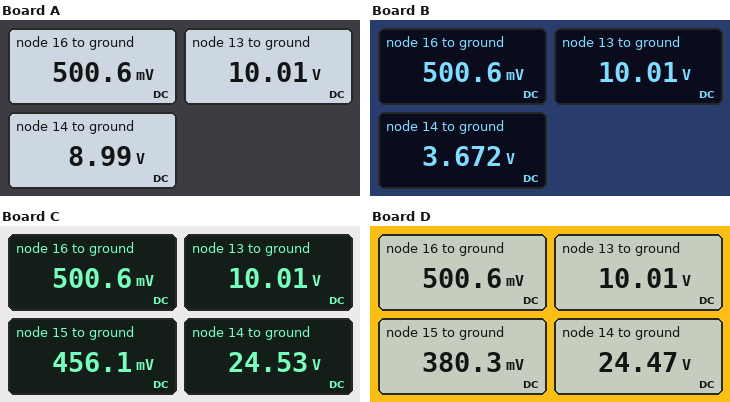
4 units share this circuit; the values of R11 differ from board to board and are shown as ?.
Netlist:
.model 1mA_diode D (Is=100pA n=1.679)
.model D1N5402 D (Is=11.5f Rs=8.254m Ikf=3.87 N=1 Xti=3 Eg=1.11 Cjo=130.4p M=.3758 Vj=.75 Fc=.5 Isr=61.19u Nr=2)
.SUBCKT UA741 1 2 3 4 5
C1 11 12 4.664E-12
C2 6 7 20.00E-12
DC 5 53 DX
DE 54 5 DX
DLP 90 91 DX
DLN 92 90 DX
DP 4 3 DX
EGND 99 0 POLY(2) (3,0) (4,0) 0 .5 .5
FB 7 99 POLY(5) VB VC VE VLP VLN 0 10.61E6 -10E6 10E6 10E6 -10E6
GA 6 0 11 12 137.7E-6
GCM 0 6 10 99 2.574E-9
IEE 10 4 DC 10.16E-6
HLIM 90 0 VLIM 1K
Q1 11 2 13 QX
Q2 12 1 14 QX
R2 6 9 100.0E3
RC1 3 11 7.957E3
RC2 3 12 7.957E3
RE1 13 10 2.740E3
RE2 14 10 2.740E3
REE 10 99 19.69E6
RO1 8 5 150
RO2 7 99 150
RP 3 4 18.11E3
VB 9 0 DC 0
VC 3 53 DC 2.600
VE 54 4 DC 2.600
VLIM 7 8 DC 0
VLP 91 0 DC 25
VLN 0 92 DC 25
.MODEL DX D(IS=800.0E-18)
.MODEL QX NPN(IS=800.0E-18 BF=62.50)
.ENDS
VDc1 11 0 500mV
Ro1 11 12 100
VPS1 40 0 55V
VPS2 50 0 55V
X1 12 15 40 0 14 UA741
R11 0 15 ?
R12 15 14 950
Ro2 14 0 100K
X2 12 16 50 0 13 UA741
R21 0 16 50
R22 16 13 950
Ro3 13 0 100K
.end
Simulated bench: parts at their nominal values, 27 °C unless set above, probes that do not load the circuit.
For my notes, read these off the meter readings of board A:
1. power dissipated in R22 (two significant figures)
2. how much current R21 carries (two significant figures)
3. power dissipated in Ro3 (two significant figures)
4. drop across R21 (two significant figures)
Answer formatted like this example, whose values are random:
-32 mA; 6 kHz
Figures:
95 mW; 10 mA; 1.0 mW; 500 mV
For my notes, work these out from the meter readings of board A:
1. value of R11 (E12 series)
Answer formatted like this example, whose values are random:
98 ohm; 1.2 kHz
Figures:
56 Ω
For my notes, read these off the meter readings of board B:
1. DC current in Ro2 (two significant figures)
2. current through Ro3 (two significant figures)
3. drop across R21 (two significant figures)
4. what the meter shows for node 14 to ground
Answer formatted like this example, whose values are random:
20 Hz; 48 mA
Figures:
37 µA; 100 µA; 500 mV; 3.672 V
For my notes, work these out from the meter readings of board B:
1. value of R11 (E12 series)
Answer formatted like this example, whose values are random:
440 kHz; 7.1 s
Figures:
150 Ω
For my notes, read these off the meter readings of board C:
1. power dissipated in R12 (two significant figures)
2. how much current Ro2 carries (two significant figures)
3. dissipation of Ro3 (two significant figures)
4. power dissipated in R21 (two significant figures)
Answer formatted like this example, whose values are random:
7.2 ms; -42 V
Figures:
610 mW; 250 µA; 1.0 mW; 5.0 mW
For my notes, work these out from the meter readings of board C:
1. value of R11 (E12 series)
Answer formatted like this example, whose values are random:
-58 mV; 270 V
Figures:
18 Ω
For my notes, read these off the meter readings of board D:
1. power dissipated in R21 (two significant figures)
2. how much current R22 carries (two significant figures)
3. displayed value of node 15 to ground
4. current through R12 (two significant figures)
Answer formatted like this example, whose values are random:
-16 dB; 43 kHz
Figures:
5.0 mW; 10 mA; 380.3 mV; 25 mA
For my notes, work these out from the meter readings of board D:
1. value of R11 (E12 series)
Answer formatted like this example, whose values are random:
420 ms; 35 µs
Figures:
15 Ω
